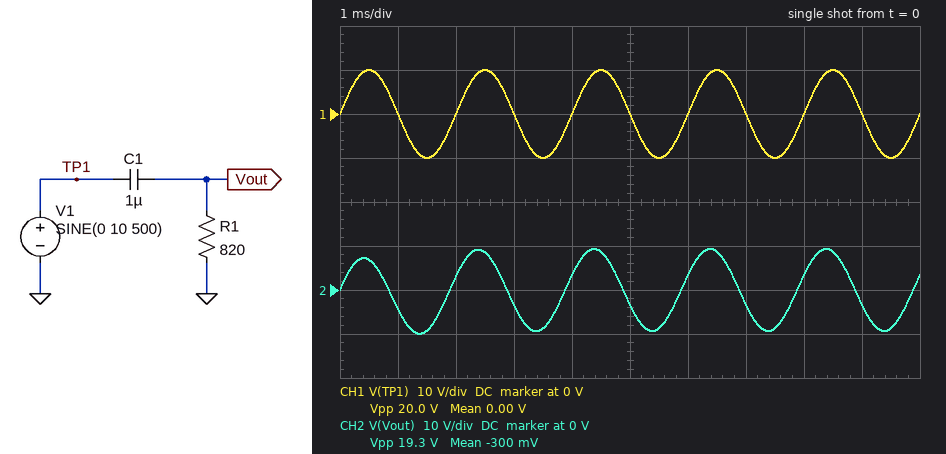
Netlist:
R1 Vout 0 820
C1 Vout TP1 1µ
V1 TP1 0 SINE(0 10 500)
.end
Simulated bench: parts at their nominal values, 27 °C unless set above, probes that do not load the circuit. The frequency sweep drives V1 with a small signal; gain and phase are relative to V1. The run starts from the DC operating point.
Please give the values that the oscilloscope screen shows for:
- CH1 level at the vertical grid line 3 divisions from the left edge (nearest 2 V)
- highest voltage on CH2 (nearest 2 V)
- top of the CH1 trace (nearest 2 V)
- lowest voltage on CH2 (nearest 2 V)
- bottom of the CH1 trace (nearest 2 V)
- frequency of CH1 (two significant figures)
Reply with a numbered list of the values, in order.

1. 0 V
2. 10 V
3. 10 V
4. -10 V
5. -10 V
6. 500 Hz
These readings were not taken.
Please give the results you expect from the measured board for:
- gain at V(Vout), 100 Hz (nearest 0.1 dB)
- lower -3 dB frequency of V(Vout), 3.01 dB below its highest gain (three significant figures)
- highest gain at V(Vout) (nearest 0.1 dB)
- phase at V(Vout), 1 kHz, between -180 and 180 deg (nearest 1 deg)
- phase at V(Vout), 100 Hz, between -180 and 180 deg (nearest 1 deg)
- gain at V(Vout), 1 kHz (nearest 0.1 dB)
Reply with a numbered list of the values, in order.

1. -6.8 dB
2. 194 Hz
3. 0 dB
4. 11 deg
5. 63 deg
6. -0.2 dB
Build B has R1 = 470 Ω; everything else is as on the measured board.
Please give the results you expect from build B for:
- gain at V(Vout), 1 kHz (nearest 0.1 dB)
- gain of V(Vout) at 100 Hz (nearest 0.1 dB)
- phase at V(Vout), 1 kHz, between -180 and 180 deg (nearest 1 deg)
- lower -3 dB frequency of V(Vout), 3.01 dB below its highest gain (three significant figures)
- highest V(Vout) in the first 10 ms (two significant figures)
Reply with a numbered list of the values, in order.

1. -0.5 dB
2. -11.0 dB
3. 19 deg
4. 339 Hz
5. 8.3 V
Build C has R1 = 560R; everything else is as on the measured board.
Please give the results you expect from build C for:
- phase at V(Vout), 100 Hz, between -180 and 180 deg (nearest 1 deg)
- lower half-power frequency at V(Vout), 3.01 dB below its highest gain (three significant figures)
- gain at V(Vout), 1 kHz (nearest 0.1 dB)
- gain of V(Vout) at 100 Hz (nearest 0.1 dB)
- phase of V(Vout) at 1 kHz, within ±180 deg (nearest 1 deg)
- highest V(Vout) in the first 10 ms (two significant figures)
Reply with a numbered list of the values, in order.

1. 71 deg
2. 284 Hz
3. -0.3 dB
4. -9.6 dB
5. 16 deg
6. 8.7 V
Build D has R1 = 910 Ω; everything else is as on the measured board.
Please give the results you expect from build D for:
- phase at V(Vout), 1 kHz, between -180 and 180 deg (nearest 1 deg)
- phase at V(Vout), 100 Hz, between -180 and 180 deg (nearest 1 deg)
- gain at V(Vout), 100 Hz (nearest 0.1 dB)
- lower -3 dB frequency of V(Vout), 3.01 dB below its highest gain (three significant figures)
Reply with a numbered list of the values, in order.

1. 10 deg
2. 60 deg
3. -6.1 dB
4. 175 Hz
